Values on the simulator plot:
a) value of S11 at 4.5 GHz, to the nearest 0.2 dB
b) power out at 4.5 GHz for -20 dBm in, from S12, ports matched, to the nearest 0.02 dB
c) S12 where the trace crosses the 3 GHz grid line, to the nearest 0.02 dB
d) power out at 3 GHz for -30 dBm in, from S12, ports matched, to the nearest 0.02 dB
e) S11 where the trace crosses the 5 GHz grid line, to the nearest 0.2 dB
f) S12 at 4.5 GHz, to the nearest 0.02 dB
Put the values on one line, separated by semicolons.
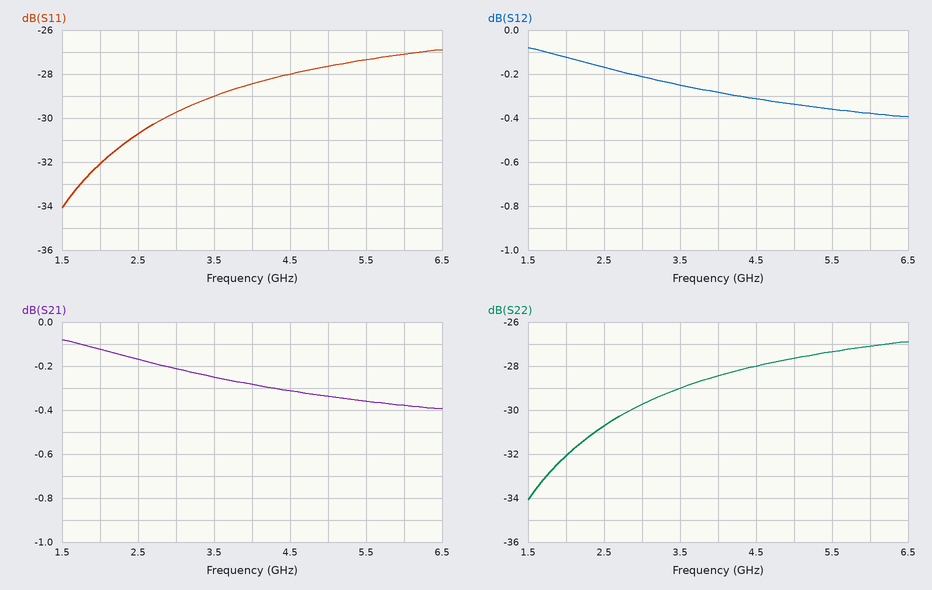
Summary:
-28.0 dB; -20.32 dBm; -0.22 dB; -30.22 dBm; -27.6 dB; -0.32 dB
